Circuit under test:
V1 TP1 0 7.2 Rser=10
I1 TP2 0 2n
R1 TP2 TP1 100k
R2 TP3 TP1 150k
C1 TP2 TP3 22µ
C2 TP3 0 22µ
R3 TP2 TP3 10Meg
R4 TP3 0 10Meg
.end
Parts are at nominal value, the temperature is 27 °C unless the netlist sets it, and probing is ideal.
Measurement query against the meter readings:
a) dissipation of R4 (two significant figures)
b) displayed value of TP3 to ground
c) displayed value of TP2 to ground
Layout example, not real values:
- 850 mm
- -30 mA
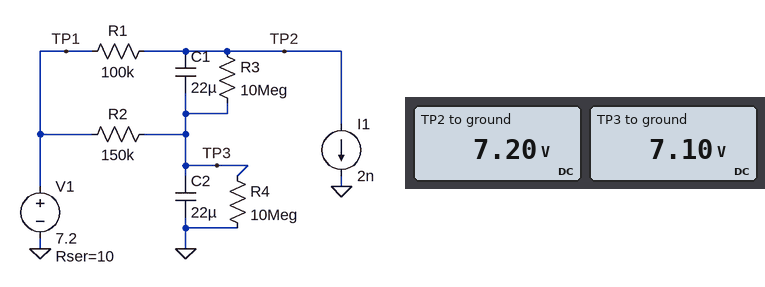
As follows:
- 5.0 µW
- 7.10 V
- 7.20 V
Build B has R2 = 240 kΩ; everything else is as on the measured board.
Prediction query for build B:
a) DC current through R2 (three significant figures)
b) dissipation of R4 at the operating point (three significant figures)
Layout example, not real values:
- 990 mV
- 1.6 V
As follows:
- 687 nA
- 4.95 µW
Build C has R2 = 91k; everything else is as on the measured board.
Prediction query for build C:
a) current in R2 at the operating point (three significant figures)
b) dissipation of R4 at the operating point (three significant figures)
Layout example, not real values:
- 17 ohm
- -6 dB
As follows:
- 707 nA
- 5.09 µW
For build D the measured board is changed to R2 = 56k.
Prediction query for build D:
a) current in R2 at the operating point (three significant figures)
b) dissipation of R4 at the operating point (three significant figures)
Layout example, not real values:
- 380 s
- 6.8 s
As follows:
- 712 nA
- 5.13 µW
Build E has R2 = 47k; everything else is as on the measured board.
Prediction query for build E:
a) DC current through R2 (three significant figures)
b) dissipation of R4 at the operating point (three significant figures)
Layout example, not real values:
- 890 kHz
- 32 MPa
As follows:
- 713 nA
- 5.14 µW
